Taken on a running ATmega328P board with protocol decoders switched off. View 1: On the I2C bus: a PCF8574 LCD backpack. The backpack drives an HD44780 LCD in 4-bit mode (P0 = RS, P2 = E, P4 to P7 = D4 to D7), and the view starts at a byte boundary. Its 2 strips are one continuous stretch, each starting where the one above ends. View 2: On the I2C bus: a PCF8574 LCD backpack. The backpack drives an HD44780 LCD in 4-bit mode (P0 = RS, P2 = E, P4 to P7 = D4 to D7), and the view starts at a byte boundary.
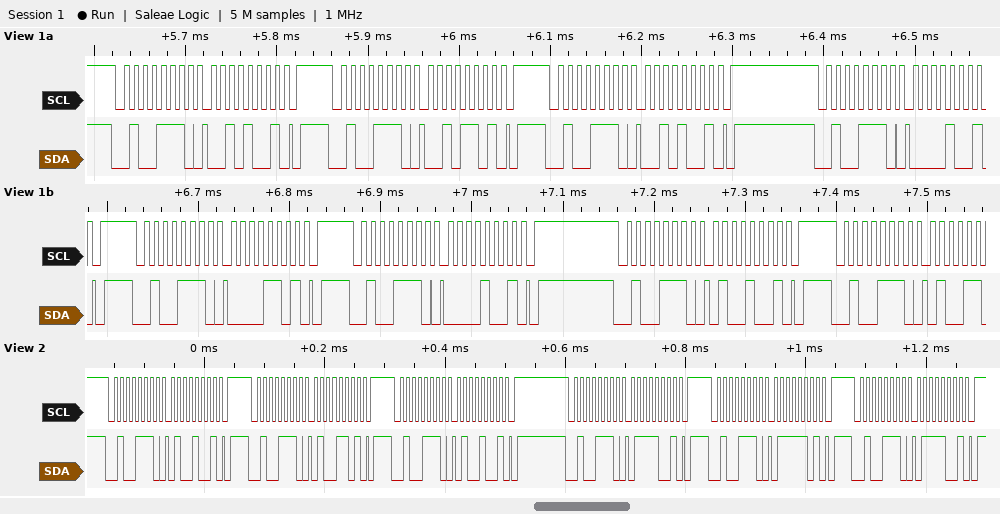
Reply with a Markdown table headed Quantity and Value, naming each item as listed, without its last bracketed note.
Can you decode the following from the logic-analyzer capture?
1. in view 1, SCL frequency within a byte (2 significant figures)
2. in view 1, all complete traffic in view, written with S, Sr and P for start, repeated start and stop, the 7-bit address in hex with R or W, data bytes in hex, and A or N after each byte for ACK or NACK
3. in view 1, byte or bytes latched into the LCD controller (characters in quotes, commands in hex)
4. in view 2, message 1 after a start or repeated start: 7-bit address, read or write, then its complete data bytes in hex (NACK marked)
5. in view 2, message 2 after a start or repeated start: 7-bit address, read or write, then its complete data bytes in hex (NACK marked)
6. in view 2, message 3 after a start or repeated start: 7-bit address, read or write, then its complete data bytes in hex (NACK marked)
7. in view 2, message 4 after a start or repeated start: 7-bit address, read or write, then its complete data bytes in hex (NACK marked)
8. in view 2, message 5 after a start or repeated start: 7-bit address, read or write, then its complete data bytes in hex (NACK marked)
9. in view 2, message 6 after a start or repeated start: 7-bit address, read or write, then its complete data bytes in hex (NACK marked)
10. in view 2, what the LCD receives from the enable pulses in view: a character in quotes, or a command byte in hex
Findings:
| Quantity | Value |
|---|---|
| in view 1, SCL frequency within a byte | 100 kHz |
| in view 1, all complete traffic in view, written with S, Sr and P for start, repeated start and stop, the 7-bit address in hex with R or W, data bytes in hex, and A or N after each byte for ACK or NACK | S 27W A 29 A P S 27W A 2D A P S 27W A 29 A P S 27W A 09 A P S 27W A 0D A P S 27W A 09 A P S 27W A 49 A P S 27W A |
| in view 1, byte or bytes latched into the LCD controller | ' ' |
| in view 2, message 1 after a start or repeated start: 7-bit address, read or write, then its complete data bytes in hex | 0x27 write: 49 |
| in view 2, message 2 after a start or repeated start: 7-bit address, read or write, then its complete data bytes in hex | 0x27 write: 4D |
| in view 2, message 3 after a start or repeated start: 7-bit address, read or write, then its complete data bytes in hex | 0x27 write: 49 |
| in view 2, message 4 after a start or repeated start: 7-bit address, read or write, then its complete data bytes in hex | 0x27 write: 79 |
| in view 2, message 5 after a start or repeated start: 7-bit address, read or write, then its complete data bytes in hex | 0x27 write: 7D |
| in view 2, message 6 after a start or repeated start: 7-bit address, read or write, then its complete data bytes in hex | 0x27 write: 79 |
| in view 2, what the LCD receives from the enable pulses in view: a character in quotes, or a command byte in hex | 'G' |
